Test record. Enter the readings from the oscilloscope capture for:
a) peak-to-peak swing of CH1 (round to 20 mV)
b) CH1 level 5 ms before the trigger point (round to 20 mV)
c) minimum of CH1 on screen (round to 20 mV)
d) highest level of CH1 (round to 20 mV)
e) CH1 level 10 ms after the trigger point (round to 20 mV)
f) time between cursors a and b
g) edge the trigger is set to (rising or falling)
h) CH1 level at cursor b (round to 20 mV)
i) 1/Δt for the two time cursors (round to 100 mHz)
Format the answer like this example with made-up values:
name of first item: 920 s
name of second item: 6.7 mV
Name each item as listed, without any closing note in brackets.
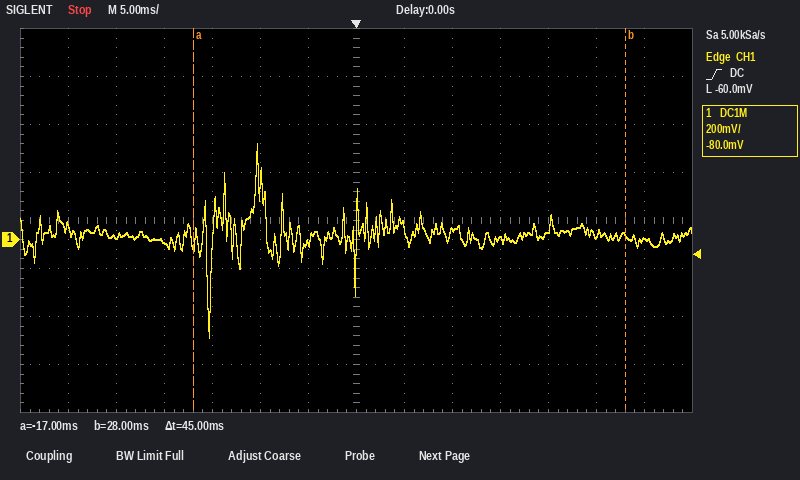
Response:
peak-to-peak swing of CH1: 800 mV
CH1 level 5 ms before the trigger point: -20 mV
minimum of CH1 on screen: -400 mV
highest level of CH1: 400 mV
CH1 level 10 ms after the trigger point: 40 mV
time between cursors a and b: 45 ms
edge the trigger is set to: rising
CH1 level at cursor b: 20 mV
1/Δt for the two time cursors: 22.2 Hz
